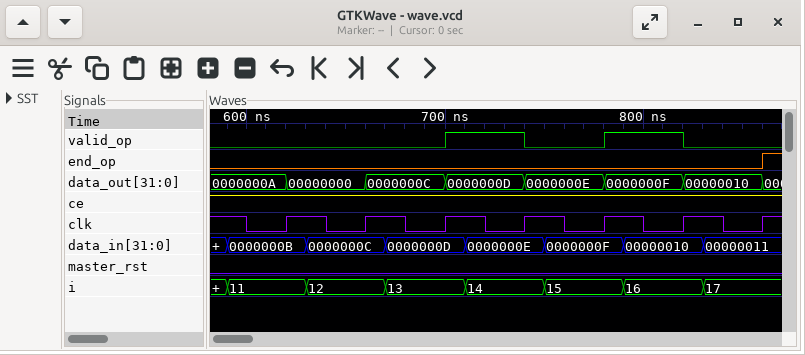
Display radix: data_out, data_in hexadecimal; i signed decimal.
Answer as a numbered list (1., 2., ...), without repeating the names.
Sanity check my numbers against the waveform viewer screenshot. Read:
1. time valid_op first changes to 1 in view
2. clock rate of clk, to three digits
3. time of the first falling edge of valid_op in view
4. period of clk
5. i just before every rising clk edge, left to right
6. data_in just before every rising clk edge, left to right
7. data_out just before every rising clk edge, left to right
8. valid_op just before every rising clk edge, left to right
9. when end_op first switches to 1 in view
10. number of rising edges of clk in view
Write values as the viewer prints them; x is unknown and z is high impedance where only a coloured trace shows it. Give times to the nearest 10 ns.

1. 700 ns
2. 25.0 MHz
3. 740 ns
4. 40 ns
5. 11, 12, 13, 14, 15, 16, 17
6. 0000000B, 0000000C, 0000000D, 0000000E, 0000000F, 00000010, 00000011
7. 0000000A, 00000000, 0000000C, 0000000D, 0000000E, 0000000F, 00000010
8. 0 0 0 1 0 1 0
9. 860 ns
10. 7
